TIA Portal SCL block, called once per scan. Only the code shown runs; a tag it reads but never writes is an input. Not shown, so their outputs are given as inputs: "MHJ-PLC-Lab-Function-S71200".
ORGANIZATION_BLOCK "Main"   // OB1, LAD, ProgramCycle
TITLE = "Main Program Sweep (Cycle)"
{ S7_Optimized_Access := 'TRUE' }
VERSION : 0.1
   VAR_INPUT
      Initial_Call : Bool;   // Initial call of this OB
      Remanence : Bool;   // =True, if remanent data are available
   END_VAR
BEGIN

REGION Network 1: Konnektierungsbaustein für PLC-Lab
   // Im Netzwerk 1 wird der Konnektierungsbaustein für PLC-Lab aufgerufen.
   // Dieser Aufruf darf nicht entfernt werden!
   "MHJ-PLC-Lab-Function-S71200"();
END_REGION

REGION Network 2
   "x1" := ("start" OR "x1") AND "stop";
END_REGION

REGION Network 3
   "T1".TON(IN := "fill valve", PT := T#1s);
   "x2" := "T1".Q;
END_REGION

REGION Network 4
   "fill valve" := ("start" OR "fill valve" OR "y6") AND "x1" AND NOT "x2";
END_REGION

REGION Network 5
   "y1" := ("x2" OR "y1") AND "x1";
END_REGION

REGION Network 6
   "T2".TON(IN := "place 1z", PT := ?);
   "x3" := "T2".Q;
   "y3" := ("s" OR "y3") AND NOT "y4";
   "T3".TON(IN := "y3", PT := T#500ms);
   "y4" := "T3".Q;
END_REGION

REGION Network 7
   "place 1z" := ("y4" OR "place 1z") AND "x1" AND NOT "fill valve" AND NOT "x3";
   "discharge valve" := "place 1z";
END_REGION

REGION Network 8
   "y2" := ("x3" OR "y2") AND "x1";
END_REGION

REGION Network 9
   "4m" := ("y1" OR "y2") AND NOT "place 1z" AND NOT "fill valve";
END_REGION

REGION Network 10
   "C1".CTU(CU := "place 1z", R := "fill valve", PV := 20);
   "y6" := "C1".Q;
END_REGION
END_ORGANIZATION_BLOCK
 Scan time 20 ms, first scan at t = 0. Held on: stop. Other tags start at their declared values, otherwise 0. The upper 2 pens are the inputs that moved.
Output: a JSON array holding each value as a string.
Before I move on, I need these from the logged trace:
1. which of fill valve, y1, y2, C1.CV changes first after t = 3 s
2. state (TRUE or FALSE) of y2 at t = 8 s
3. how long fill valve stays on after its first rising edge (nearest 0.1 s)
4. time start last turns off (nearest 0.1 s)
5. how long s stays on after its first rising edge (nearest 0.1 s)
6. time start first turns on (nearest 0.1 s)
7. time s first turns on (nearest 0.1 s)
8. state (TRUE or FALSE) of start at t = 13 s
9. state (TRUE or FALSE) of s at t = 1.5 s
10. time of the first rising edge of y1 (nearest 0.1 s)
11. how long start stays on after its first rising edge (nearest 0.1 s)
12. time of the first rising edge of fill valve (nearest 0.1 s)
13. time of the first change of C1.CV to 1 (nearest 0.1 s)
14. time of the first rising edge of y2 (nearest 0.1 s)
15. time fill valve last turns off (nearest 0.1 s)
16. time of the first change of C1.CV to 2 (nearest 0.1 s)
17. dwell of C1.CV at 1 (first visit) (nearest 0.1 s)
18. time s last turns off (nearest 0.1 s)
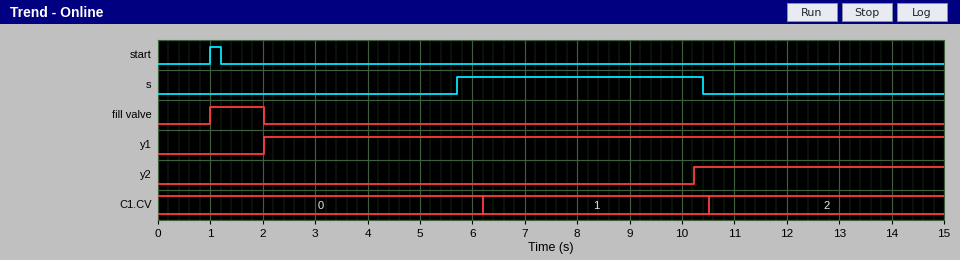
["C1.CV", "FALSE", "1.0 s", "1.2 s", "4.7 s", "1.0 s", "5.7 s", "FALSE", "FALSE", "2.0 s", "0.2 s", "1.0 s", "6.2 s", "10.2 s", "2.0 s", "10.5 s", "4.3 s", "10.4 s"]
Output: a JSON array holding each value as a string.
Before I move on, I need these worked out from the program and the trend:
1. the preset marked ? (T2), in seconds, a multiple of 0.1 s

["4.0 s"]
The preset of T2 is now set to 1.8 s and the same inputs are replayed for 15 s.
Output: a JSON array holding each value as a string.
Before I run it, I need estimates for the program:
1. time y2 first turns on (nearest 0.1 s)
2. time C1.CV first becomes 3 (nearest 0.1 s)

["8.0 s", "10.5 s"]
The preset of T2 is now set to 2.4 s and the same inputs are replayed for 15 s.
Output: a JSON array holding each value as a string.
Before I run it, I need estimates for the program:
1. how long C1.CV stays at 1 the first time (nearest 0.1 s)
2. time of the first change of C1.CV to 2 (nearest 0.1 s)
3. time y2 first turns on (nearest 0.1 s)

["2.7 s", "8.9 s", "8.6 s"]
